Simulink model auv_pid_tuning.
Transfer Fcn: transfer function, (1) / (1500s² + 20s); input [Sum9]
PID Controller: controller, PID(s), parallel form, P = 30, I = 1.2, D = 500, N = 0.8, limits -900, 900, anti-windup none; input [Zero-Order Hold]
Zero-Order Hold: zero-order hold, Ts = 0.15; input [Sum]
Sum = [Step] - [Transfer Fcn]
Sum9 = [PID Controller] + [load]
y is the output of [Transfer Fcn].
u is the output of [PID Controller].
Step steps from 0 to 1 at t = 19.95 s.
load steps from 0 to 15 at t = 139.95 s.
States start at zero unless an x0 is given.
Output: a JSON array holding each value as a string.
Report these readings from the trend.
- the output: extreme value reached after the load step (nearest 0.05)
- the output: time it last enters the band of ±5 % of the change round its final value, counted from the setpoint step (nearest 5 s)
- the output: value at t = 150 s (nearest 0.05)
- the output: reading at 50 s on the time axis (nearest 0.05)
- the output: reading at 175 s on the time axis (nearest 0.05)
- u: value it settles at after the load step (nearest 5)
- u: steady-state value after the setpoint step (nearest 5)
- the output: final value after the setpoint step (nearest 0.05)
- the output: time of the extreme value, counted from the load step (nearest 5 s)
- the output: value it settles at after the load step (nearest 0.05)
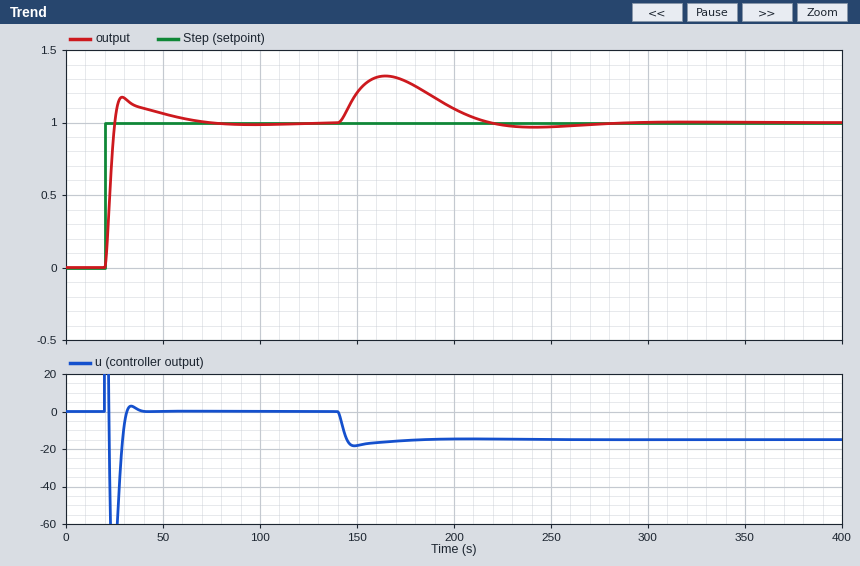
["1.30", "35 s", "1.20", "1.05", "1.30", "-15", "0", "1.00", "25 s", "1.00"]
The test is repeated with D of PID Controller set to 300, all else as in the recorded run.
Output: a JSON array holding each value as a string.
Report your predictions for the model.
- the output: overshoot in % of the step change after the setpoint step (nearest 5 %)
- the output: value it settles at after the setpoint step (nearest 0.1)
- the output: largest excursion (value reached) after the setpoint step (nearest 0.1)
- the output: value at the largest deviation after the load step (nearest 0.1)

["30 %", "1.0", "1.3", "1.4"]
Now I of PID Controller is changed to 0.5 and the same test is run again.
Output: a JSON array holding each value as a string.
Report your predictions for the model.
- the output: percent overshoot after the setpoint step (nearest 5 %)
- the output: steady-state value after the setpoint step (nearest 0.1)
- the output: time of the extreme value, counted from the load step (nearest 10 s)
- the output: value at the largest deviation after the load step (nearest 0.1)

["15 %", "1.0", "30 s", "1.4"]
